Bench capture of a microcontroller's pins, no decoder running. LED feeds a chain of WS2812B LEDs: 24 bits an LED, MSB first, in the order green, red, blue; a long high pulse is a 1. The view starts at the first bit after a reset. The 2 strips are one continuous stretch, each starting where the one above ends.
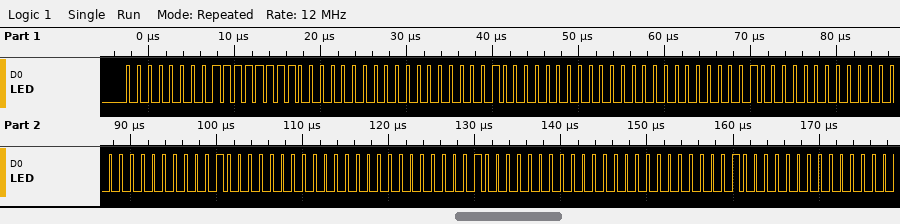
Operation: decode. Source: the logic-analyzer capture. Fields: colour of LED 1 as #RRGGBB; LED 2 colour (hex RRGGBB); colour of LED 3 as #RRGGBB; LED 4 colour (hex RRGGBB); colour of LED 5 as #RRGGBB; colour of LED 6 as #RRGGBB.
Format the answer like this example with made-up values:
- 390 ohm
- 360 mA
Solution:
- #FF0000
- #200000
- #200000
- #200000
- #200000
- #200000
